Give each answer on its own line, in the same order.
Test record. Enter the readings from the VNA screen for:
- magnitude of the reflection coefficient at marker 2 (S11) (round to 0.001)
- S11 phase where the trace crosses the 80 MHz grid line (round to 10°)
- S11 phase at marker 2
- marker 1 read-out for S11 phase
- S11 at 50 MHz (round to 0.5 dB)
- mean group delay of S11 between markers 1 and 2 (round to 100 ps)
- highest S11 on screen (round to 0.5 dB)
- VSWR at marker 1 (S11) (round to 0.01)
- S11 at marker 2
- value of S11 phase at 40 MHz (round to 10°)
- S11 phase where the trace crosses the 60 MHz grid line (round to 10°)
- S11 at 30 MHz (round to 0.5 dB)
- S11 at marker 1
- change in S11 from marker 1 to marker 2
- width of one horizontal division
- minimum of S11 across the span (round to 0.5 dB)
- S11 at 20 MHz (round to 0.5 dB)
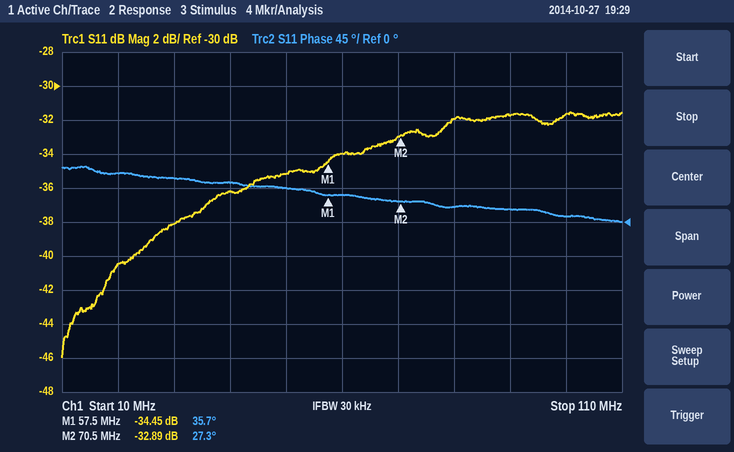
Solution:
0.023
20°
27.3°
35.7°
-35.0 dB
1.8 ns
-31.5 dB
1.04
-32.89 dB
50°
40°
-38.0 dB
-34.45 dB
1.56 dB
10 MHz
-46.0 dB
-40.5 dB
